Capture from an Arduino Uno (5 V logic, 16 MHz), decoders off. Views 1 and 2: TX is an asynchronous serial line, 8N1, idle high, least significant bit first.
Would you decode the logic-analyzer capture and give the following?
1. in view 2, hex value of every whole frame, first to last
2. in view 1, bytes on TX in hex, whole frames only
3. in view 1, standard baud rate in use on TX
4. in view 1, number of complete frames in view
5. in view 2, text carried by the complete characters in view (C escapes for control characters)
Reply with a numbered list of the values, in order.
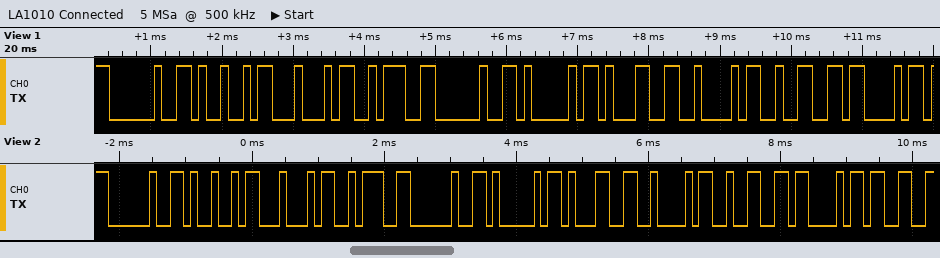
1. 20 49 44 3A 20 41 31 42 32 43 33
2. 0x20 0x49 0x44 0x3A 0x20 0x41 0x31 0x42 0x32 0x43
3. 9600 baud
4. 10
5. " ID: A1B2C3"
